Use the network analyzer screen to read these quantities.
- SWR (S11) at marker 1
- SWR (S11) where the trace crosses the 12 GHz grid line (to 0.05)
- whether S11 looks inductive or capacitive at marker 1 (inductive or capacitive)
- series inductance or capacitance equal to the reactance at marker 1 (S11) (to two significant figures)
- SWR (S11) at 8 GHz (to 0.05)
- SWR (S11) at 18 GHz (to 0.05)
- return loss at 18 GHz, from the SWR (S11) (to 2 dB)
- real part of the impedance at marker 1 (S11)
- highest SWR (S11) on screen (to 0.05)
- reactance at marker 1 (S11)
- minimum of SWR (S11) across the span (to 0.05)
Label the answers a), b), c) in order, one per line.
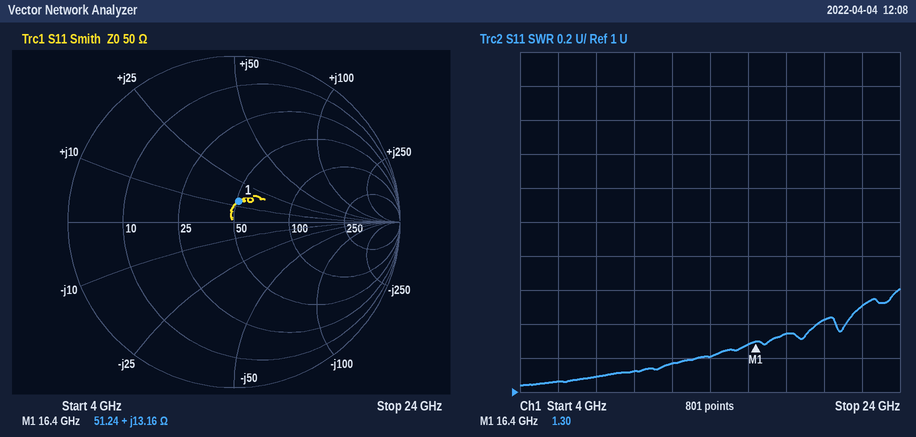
a) 1.30
b) 1.15
c) inductive
d) 130 pH
e) 1.10
f) 1.35
g) 16 dB
h) 51.24 Ω
i) 1.60
j) +13.16 Ω
k) 1.05
